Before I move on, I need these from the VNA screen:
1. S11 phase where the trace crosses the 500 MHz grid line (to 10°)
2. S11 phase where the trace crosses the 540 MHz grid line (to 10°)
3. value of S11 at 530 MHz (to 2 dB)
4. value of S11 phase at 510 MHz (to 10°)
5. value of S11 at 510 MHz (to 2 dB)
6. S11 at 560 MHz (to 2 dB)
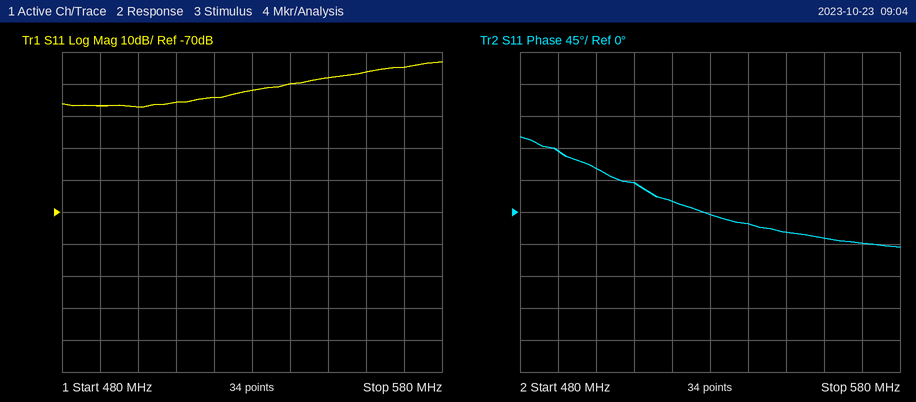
60°
-20°
-32 dB
40°
-36 dB
-26 dB
